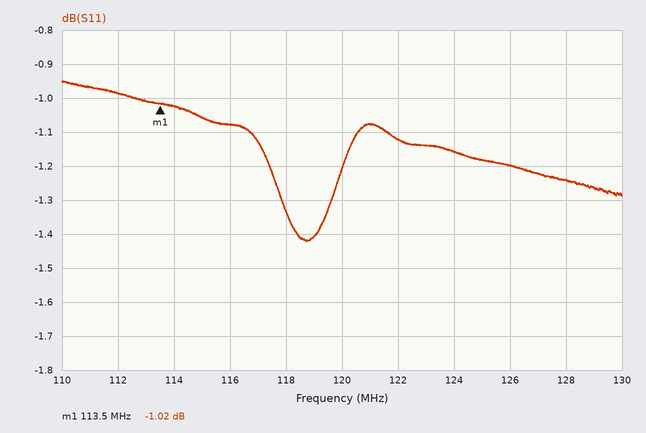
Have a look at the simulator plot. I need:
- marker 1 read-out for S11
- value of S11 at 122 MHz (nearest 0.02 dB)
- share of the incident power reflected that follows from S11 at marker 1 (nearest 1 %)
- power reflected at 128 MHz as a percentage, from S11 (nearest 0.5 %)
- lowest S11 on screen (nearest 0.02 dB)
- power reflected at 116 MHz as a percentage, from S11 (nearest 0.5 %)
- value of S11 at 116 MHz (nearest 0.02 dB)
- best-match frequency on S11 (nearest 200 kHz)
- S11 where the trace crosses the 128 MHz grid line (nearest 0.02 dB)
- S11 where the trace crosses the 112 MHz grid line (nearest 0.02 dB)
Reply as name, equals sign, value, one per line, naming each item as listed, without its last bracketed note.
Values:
marker 1 read-out for S11 = -1.02 dB
value of S11 at 122 MHz = -1.12 dB
share of the incident power reflected that follows from S11 at marker 1 = 79 %
power reflected at 128 MHz as a percentage, from S11 = 75.0 %
lowest S11 on screen = -1.42 dB
power reflected at 116 MHz as a percentage, from S11 = 78.0 %
value of S11 at 116 MHz = -1.08 dB
best-match frequency on S11 = 118.8 MHz
S11 where the trace crosses the 128 MHz grid line = -1.24 dB
S11 where the trace crosses the 112 MHz grid line = -0.98 dB
